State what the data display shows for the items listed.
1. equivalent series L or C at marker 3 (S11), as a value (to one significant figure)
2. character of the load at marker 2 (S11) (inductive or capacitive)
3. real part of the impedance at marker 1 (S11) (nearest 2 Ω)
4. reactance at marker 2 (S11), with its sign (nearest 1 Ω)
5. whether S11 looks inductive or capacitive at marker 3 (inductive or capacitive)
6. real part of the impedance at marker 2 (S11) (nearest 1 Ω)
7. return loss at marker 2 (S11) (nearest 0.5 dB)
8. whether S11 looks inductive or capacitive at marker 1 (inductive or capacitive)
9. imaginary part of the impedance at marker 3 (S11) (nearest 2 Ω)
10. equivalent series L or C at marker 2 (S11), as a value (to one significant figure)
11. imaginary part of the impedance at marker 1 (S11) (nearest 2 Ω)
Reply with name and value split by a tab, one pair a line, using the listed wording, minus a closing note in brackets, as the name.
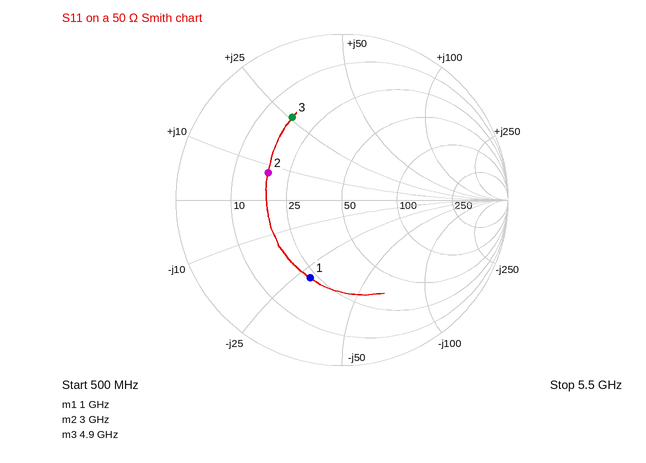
equivalent series L or C at marker 3 (S11), as a value	800 pH
character of the load at marker 2 (S11)	inductive
real part of the impedance at marker 1 (S11)	22 Ω
reactance at marker 2 (S11), with its sign	+8 Ω
whether S11 looks inductive or capacitive at marker 3	inductive
real part of the impedance at marker 2 (S11)	18 Ω
return loss at marker 2 (S11)	6.5 dB
whether S11 looks inductive or capacitive at marker 1	capacitive
imaginary part of the impedance at marker 3 (S11)	+26 Ω
equivalent series L or C at marker 2 (S11), as a value	400 pH
imaginary part of the impedance at marker 1 (S11)	-28 Ω
